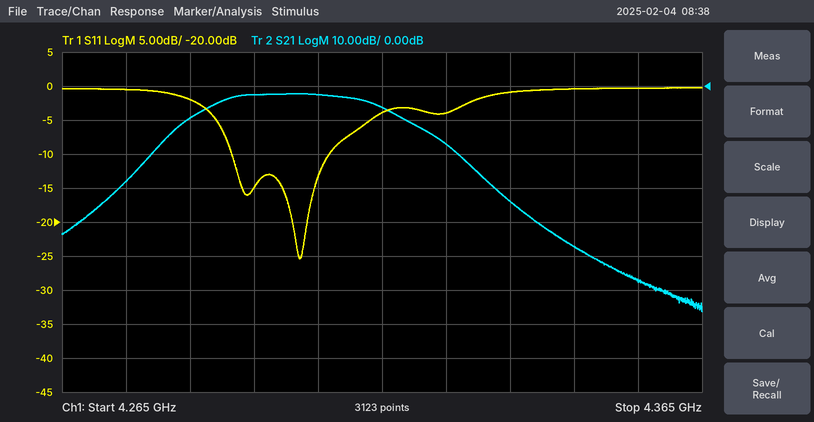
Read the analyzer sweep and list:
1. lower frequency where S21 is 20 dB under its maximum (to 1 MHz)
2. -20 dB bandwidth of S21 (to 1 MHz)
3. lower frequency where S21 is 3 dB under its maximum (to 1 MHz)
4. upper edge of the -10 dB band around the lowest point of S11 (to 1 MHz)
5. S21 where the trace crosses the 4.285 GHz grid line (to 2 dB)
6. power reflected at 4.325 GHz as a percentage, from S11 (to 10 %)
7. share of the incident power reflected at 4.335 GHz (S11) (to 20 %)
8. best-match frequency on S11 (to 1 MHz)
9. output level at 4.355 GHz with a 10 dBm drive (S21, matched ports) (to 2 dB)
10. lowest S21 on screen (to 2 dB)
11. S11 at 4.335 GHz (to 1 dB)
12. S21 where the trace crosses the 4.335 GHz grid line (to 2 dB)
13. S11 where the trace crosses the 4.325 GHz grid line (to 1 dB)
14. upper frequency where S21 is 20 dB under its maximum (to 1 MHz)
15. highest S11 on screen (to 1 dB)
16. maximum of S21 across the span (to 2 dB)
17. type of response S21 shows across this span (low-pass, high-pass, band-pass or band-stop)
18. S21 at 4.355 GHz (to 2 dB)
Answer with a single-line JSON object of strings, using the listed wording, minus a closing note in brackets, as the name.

{"lower frequency where S21 is 20 dB under its maximum": "4.278 GHz", "-20 dB bandwidth of S21": "50 MHz", "lower frequency where S21 is 3 dB under its maximum": "4.289 GHz", "upper edge of the -10 dB band around the lowest point of S11": "4.307 GHz", "S21 where the trace crosses the 4.285 GHz grid line": "-10 dB", "power reflected at 4.325 GHz as a percentage, from S11": "40 %", "share of the incident power reflected at 4.335 GHz (S11)": "80 %", "best-match frequency on S11": "4.302 GHz", "output level at 4.355 GHz with a 10 dBm drive (S21, matched ports)": "-48 dBm", "lowest S21 on screen": "-66 dB", "S11 at 4.335 GHz": "-1 dB", "S21 where the trace crosses the 4.335 GHz grid line": "-34 dB", "S11 where the trace crosses the 4.325 GHz grid line": "-4 dB", "upper frequency where S21 is 20 dB under its maximum": "4.328 GHz", "highest S11 on screen": "0 dB", "maximum of S21 across the span": "-2 dB", "type of response S21 shows across this span": "band-pass", "S21 at 4.355 GHz": "-58 dB"}
